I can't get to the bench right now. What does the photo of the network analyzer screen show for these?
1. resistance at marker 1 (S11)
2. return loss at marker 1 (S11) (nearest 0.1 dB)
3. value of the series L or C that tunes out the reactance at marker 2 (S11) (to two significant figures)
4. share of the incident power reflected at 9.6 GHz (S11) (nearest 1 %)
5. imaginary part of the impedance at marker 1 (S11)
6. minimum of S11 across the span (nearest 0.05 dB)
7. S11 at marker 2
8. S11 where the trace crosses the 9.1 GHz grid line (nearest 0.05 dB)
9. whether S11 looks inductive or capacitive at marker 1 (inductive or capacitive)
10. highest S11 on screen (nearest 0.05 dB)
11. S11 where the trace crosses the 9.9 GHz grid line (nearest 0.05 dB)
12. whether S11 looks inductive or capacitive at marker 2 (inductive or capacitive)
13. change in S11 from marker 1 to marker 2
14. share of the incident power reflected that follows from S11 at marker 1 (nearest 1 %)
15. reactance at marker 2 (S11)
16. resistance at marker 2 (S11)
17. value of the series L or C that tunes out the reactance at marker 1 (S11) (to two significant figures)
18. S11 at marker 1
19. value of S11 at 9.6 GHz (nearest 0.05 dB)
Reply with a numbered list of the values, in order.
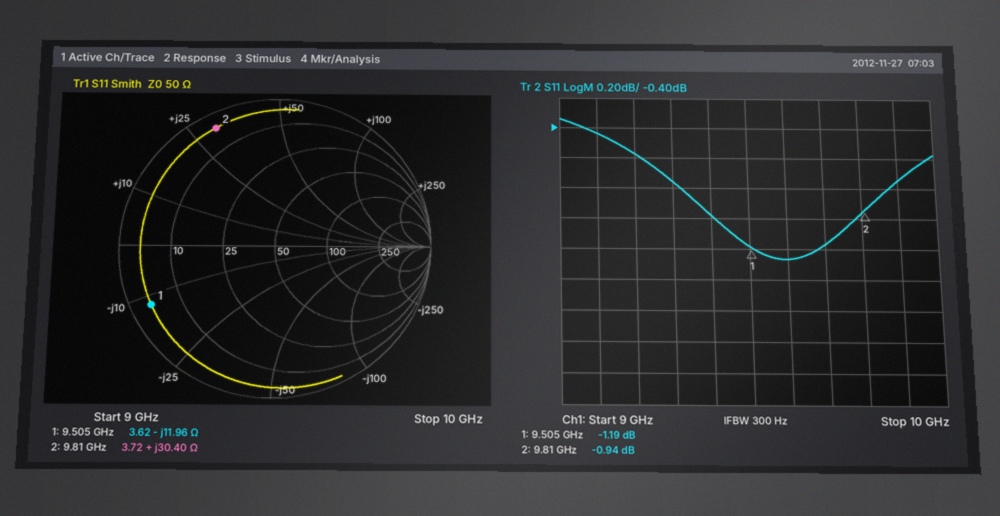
1. 3.62 Ω
2. 1.2 dB
3. 530 fF
4. 75 %
5. -11.96 Ω
6. -1.25 dB
7. -0.94 dB
8. -0.45 dB
9. capacitive
10. -0.35 dB
11. -0.75 dB
12. inductive
13. 0.25 dB
14. 76 %
15. +30.40 Ω
16. 3.72 Ω
17. 200 pH
18. -1.19 dB
19. -1.25 dB
